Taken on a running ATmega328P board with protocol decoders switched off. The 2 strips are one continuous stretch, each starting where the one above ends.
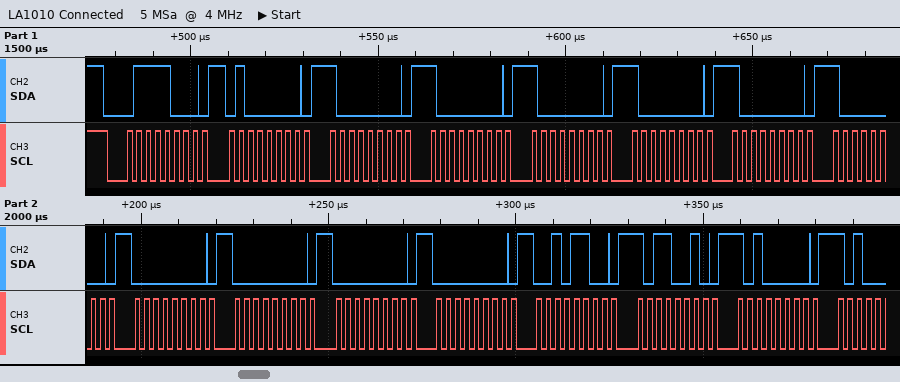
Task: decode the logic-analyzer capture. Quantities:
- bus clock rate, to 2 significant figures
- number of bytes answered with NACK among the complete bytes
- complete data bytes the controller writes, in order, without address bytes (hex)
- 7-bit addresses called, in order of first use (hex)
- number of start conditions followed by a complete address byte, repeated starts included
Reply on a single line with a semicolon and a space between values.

400 kHz; 0; 40 80 80 80 80 80 80 00 00 00 00 2C B2 A0; 0x3C; 1
